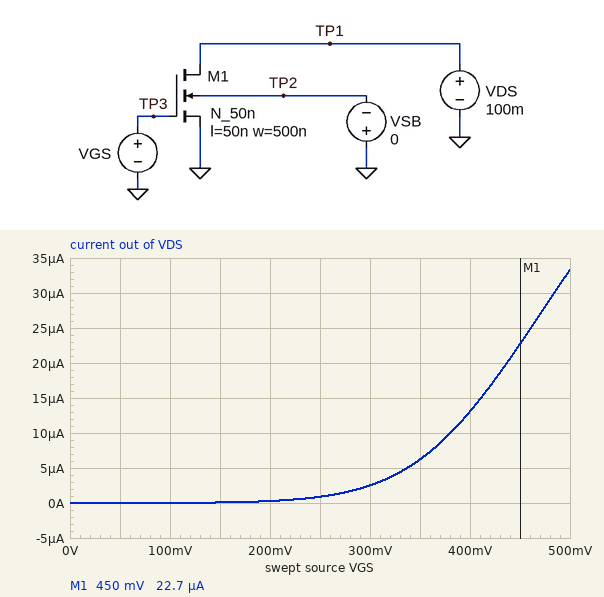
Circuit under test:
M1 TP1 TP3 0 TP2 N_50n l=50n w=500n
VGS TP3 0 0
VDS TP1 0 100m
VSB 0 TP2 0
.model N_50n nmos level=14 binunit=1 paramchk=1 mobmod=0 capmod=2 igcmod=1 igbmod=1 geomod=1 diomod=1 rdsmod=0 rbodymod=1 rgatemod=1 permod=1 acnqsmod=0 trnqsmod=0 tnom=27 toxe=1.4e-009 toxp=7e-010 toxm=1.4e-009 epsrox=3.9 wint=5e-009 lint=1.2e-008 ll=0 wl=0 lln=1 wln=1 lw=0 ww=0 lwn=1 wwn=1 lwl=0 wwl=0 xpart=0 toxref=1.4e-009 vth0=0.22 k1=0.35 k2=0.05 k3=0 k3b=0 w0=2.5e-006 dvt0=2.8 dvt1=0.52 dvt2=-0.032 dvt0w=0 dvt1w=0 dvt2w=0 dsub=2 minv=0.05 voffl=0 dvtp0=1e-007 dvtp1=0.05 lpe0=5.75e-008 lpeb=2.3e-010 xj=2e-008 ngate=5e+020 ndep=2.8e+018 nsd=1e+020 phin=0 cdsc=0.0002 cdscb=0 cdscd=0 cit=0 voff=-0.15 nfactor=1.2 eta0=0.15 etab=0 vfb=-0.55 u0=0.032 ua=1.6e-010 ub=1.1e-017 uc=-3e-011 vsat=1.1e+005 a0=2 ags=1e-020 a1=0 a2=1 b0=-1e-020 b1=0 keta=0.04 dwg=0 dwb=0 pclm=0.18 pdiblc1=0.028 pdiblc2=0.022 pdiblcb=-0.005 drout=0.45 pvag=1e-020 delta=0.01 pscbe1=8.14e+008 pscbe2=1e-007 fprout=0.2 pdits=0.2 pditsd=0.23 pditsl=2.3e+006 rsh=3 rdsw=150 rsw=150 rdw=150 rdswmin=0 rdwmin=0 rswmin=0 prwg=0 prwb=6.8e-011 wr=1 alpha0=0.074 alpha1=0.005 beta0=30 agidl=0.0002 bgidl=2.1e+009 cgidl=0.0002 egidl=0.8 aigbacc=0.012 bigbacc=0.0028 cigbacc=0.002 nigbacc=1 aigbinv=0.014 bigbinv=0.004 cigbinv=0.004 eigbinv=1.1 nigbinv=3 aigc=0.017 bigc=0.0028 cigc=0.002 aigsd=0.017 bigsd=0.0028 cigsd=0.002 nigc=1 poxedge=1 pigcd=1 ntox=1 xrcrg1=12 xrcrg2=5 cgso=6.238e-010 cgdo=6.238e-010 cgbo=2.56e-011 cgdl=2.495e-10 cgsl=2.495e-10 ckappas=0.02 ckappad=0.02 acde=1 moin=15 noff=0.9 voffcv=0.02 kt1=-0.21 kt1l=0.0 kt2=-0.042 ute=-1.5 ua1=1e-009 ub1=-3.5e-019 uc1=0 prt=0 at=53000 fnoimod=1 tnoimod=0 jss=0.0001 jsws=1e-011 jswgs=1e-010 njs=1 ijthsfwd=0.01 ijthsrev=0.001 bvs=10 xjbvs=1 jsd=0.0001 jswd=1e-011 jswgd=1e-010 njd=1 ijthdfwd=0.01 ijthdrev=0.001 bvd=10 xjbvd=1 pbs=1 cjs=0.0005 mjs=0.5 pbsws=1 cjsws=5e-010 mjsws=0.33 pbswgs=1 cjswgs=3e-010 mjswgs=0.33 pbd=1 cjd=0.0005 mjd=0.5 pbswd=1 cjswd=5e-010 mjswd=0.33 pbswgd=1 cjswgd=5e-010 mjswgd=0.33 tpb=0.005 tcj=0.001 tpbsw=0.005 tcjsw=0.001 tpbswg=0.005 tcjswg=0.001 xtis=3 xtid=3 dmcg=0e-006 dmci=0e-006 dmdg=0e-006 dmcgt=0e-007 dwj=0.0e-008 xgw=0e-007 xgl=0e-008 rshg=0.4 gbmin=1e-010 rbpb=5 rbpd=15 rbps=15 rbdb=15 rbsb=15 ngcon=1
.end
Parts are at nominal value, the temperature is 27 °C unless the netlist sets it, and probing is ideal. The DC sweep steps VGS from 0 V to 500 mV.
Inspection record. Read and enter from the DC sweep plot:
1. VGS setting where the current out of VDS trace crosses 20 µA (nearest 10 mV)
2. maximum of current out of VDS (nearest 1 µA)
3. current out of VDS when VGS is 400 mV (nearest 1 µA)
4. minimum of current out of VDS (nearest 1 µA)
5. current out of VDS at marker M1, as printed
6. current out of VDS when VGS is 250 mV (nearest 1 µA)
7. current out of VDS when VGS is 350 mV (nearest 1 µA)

440 mV
33 µA
13 µA
0 A
22.7 µA
1 µA
6 µA
